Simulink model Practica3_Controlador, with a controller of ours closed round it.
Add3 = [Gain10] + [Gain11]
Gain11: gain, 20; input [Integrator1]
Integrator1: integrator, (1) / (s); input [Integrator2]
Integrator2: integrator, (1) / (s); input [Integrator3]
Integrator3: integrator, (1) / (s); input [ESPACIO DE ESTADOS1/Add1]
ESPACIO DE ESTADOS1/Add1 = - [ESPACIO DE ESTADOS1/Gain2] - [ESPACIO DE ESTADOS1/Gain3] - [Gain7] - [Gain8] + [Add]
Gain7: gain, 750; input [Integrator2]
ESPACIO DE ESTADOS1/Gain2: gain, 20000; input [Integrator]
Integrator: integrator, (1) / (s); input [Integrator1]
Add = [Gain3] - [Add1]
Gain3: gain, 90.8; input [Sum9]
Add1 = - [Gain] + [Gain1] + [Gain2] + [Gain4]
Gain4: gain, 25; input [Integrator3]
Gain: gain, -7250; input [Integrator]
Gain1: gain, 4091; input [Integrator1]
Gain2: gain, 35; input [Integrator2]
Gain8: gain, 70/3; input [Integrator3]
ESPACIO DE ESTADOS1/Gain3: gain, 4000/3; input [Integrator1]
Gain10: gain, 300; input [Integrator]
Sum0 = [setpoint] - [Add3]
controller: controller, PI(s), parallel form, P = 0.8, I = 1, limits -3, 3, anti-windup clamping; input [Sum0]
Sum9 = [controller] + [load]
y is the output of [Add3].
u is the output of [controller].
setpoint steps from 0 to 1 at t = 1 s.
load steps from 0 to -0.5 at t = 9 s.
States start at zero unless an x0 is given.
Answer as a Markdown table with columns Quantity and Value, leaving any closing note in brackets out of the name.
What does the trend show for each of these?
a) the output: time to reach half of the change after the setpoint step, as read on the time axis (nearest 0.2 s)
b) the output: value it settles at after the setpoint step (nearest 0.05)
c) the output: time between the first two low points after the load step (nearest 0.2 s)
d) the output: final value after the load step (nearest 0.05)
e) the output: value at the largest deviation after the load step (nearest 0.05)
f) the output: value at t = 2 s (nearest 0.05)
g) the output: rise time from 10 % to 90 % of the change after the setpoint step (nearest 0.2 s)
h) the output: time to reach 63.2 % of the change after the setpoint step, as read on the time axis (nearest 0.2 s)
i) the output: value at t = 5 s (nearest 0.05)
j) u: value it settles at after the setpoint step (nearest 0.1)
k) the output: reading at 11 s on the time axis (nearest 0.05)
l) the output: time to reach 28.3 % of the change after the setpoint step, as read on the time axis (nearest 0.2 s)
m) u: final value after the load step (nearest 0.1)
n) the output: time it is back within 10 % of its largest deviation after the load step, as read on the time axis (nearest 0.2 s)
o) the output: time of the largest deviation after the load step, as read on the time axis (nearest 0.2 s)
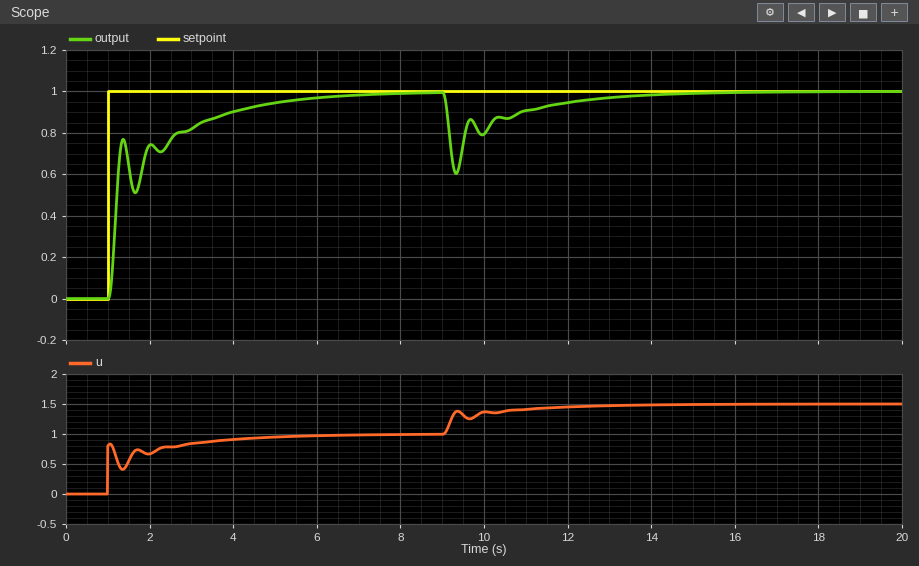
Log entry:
| Quantity | Value |
|---|---|
| the output: time to reach half of the change after the setpoint step, as read on the time axis | 1.2 s |
| the output: value it settles at after the setpoint step | 1.00 |
| the output: time between the first two low points after the load step | 0.6 s |
| the output: final value after the load step | 1.00 |
| the output: value at the largest deviation after the load step | 0.60 |
| the output: value at t = 2 s | 0.75 |
| the output: rise time from 10 % to 90 % of the change after the setpoint step | 2.8 s |
| the output: time to reach 63.2 % of the change after the setpoint step, as read on the time axis | 1.2 s |
| the output: value at t = 5 s | 0.95 |
| u: value it settles at after the setpoint step | 1.0 |
| the output: reading at 11 s on the time axis | 0.90 |
| the output: time to reach 28.3 % of the change after the setpoint step, as read on the time axis | 1.2 s |
| u: final value after the load step | 1.5 |
| the output: time it is back within 10 % of its largest deviation after the load step, as read on the time axis | 12.6 s |
| the output: time of the largest deviation after the load step, as read on the time axis | 9.4 s |
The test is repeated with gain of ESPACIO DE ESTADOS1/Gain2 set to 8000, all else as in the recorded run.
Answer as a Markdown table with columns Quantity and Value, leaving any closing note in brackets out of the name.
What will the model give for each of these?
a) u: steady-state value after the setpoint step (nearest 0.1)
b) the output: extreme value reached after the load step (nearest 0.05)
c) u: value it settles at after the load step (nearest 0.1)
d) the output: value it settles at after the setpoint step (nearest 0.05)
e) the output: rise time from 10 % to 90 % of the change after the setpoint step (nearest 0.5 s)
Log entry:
| Quantity | Value |
|---|---|
| u: steady-state value after the setpoint step | 0.6 |
| the output: extreme value reached after the load step | 0.55 |
| u: value it settles at after the load step | 1.1 |
| the output: value it settles at after the setpoint step | 1.00 |
| the output: rise time from 10 % to 90 % of the change after the setpoint step | 1.5 s |
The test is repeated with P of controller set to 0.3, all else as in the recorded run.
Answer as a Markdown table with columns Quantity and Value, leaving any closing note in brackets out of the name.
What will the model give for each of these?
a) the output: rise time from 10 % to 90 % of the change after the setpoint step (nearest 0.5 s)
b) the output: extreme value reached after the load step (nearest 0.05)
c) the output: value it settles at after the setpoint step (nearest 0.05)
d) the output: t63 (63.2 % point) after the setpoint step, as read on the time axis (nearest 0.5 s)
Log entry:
| Quantity | Value |
|---|---|
| the output: rise time from 10 % to 90 % of the change after the setpoint step | 2.5 s |
| the output: extreme value reached after the load step | 0.50 |
| the output: value it settles at after the setpoint step | 1.00 |
| the output: t63 (63.2 % point) after the setpoint step, as read on the time axis | 2.0 s |
